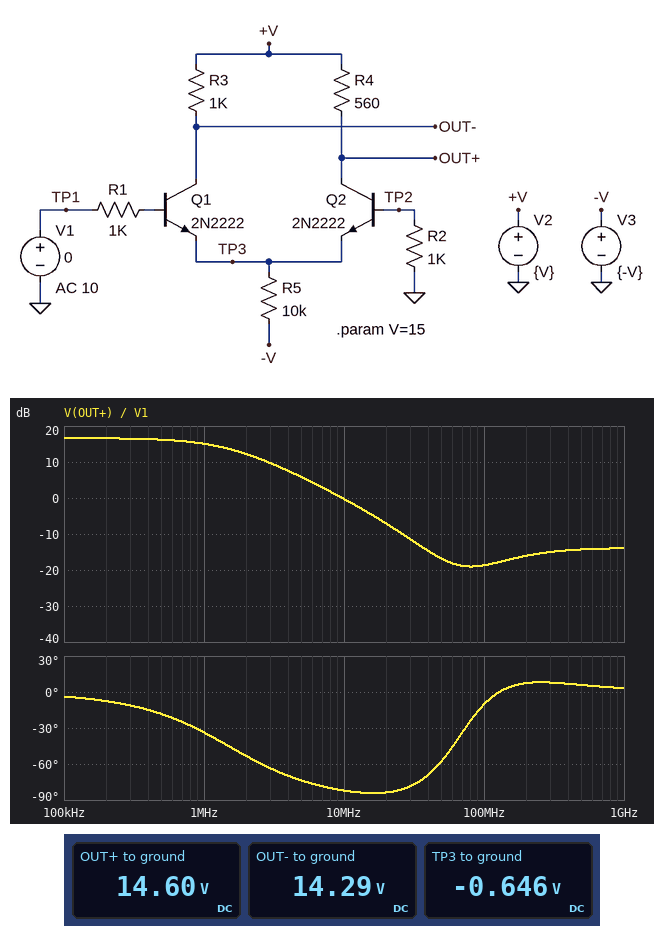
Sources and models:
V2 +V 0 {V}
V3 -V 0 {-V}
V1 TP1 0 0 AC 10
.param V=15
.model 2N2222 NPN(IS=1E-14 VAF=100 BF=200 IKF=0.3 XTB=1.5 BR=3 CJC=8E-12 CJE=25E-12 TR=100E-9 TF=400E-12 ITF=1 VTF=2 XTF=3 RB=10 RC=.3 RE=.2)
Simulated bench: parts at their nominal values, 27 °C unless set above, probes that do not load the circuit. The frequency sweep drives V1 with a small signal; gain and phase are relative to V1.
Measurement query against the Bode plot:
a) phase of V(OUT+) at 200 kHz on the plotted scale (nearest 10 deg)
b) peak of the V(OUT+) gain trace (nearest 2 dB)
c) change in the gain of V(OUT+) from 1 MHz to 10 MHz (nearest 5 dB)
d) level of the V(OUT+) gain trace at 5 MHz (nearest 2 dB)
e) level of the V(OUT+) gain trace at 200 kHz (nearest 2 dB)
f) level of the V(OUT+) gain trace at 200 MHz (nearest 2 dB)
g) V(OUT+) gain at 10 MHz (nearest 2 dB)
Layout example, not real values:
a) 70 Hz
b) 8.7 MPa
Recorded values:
a) -10 deg
b) 16 dB
c) -15 dB
d) 6 dB
e) 16 dB
f) -16 dB
g) 0 dB
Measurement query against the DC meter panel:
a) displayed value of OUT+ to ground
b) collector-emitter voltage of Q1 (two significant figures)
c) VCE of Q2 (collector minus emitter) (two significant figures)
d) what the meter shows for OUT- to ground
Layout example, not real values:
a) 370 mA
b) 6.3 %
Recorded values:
a) 14.60 V
b) 15 V
c) 15 V
d) 14.29 V
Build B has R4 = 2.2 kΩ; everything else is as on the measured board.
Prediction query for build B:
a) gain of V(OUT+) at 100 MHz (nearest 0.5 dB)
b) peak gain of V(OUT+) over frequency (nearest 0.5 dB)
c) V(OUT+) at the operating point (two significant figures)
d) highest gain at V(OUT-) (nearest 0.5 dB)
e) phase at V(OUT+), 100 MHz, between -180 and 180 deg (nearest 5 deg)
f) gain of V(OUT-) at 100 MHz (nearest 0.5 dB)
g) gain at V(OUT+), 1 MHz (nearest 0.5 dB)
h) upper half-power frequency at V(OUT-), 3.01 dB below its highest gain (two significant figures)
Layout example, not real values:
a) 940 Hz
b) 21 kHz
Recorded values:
a) -14.0 dB
b) 28.5 dB
c) 13 V
d) 21.5 dB
e) -20 deg
f) -9.0 dB
g) 25.0 dB
h) 940 kHz
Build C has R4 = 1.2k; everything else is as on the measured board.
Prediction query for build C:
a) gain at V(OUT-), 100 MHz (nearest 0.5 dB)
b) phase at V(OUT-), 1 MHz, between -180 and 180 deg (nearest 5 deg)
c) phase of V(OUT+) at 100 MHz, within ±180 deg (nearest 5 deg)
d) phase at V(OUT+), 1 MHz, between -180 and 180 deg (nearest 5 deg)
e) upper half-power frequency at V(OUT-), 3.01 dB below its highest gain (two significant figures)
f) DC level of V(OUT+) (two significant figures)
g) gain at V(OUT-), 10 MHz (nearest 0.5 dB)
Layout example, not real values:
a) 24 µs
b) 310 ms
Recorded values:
a) -9.0 dB
b) 140 deg
c) -15 deg
d) -40 deg
e) 1.2 MHz
f) 14 V
g) 4.0 dB
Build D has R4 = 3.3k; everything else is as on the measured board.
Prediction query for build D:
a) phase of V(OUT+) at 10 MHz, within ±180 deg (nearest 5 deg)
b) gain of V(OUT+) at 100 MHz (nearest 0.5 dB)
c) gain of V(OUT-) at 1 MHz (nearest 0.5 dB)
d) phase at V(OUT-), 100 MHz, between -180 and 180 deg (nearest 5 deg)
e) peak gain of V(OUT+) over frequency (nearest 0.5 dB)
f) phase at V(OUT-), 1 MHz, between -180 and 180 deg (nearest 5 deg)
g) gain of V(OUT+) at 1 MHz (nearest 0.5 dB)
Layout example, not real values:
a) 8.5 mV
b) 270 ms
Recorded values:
a) -95 deg
b) -13.5 dB
c) 17.0 dB
d) 25 deg
e) 32.0 dB
f) 130 deg
g) 27.5 dB
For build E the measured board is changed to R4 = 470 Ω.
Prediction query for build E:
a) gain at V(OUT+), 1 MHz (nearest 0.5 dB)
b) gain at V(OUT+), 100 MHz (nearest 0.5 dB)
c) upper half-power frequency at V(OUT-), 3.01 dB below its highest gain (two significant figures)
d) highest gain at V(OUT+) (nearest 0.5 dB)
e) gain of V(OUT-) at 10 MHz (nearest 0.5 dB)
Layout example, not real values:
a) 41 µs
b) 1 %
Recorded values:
a) 13.5 dB
b) -19.5 dB
c) 1.6 MHz
d) 15.0 dB
e) 5.5 dB
